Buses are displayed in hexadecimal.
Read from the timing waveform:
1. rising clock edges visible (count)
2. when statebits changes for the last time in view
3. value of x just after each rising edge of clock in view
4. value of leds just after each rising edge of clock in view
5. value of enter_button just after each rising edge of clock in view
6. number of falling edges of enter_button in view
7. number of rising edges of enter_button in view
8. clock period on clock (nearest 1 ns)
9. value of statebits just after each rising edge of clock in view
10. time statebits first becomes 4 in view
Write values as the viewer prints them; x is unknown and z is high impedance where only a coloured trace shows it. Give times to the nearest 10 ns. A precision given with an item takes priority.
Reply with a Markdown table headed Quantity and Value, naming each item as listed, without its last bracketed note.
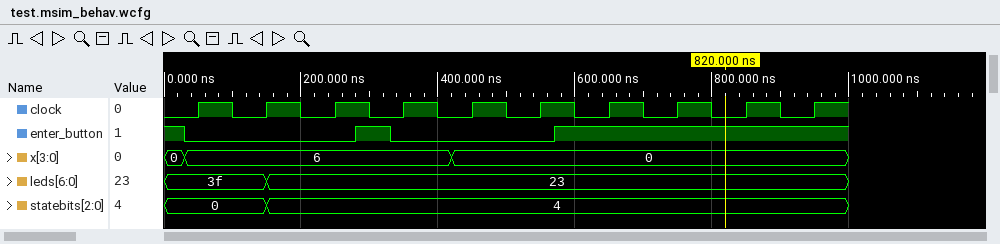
| Quantity | Value |
|---|---|
| rising clock edges visible | 10 |
| when statebits changes for the last time in view | 150 ns |
| value of x just after each rising edge of clock in view | 6, 6, 6, 6, 0, 0, 0, 0, 0, 0 |
| value of leds just after each rising edge of clock in view | 3f, 23, 23, 23, 23, 23, 23, 23, 23, 23 |
| value of enter_button just after each rising edge of clock in view | 0 0 0 0 0 0 1 1 1 1 |
| number of falling edges of enter_button in view | 2 |
| number of rising edges of enter_button in view | 2 |
| clock period on clock | 100 ns |
| value of statebits just after each rising edge of clock in view | 0, 4, 4, 4, 4, 4, 4, 4, 4, 4 |
| time statebits first becomes 4 in view | 150 ns |
